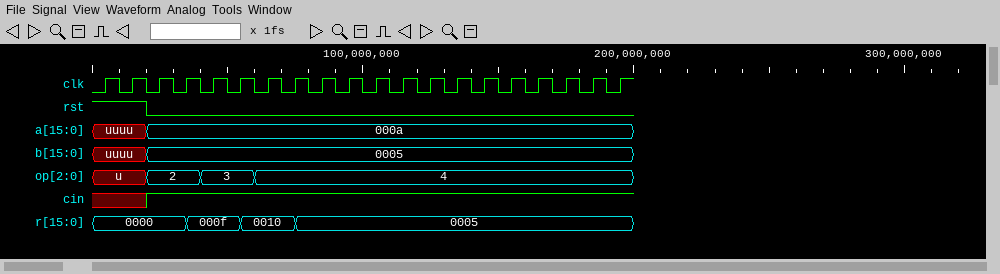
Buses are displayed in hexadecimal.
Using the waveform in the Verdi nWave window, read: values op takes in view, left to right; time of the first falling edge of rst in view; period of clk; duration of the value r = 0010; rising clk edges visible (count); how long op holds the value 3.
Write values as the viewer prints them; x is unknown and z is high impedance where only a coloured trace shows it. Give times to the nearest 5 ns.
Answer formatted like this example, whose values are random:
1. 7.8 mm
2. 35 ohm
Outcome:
1. u, 2, 3, 4
2. 20 ns
3. 10 ns
4. 20 ns
5. 20
6. 20 ns
